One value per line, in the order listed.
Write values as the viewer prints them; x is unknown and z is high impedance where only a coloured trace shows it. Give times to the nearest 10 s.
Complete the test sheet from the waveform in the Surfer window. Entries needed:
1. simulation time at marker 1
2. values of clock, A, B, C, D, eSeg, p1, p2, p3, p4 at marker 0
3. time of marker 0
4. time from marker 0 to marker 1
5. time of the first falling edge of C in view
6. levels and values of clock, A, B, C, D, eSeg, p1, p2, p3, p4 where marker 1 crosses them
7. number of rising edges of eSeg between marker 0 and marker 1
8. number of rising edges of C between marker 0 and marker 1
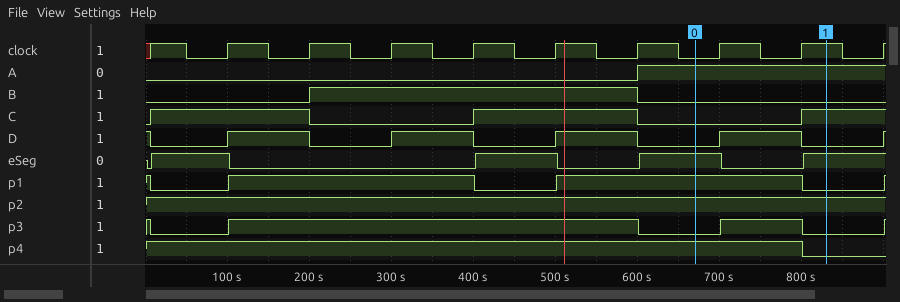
830 s
clock=0, A=1, B=0, C=0, D=0, eSeg=1, p1=1, p2=1, p3=0, p4=1
670 s
160 s
200 s
clock=1, A=1, B=0, C=1, D=0, eSeg=1, p1=0, p2=1, p3=0, p4=0
1
1
